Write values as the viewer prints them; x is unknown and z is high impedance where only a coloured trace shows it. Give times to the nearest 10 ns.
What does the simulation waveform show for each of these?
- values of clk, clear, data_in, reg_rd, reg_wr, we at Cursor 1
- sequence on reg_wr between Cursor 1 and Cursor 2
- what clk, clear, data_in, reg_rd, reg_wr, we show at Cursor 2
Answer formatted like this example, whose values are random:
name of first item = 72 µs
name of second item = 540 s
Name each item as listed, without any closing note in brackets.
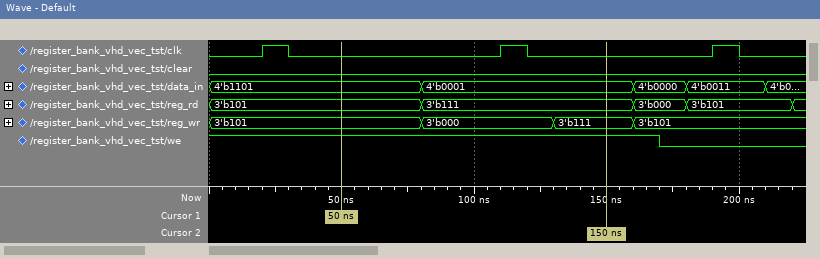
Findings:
values of clk, clear, data_in, reg_rd, reg_wr, we at Cursor 1 = clk=0, clear=0, data_in=4'b1101, reg_rd=3'b101, reg_wr=3'b101, we=1
sequence on reg_wr between Cursor 1 and Cursor 2 = 3'b101, 3'b000, 3'b111
what clk, clear, data_in, reg_rd, reg_wr, we show at Cursor 2 = clk=0, clear=0, data_in=4'b0001, reg_rd=3'b111, reg_wr=3'b111, we=1
